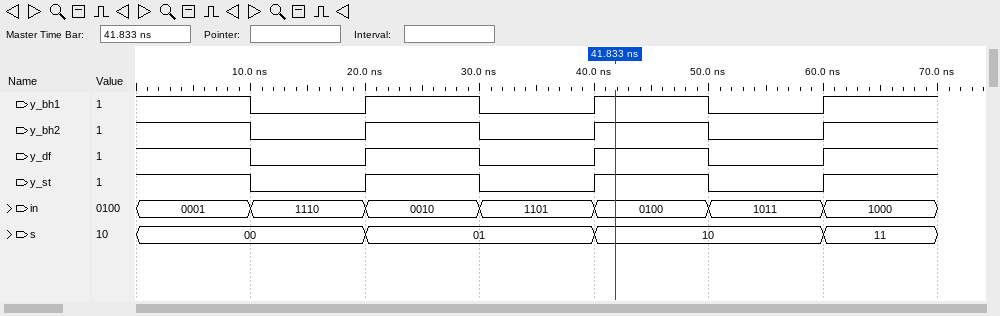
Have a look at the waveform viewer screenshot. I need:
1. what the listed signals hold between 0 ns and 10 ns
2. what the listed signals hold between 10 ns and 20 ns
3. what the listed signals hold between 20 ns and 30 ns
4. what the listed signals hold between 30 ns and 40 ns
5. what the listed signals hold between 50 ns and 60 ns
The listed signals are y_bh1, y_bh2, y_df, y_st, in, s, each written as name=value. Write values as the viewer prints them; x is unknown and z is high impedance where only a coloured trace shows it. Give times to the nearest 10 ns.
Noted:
y_bh1=1, y_bh2=1, y_df=1, y_st=1, in=0001, s=00
y_bh1=0, y_bh2=0, y_df=0, y_st=0, in=1110, s=00
y_bh1=1, y_bh2=1, y_df=1, y_st=1, in=0010, s=01
y_bh1=0, y_bh2=0, y_df=0, y_st=0, in=1101, s=01
y_bh1=0, y_bh2=0, y_df=0, y_st=0, in=1011, s=10
